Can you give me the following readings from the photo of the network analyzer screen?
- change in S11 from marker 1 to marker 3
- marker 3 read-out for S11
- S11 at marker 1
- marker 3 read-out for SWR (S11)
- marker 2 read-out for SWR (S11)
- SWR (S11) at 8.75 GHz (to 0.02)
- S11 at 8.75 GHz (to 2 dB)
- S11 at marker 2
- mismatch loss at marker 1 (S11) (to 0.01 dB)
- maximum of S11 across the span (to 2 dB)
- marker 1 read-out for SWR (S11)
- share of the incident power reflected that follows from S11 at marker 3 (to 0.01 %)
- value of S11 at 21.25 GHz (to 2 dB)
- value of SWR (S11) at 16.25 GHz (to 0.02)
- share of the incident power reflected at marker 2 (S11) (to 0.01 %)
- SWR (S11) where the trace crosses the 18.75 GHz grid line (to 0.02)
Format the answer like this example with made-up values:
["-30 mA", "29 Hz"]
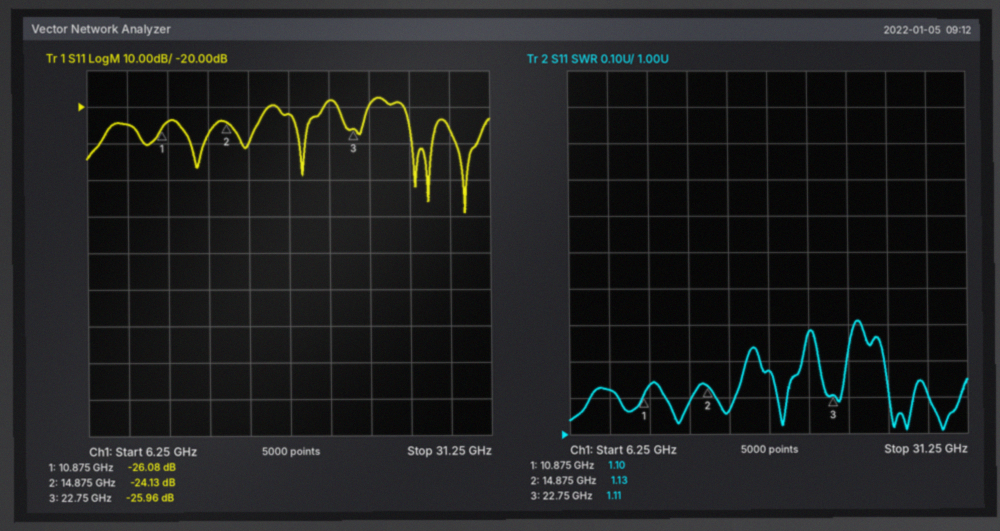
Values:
["0.12 dB", "-25.96 dB", "-26.08 dB", "1.11", "1.13", "1.12", "-24 dB", "-24.13 dB", "0.01 dB", "-18 dB", "1.10", "0.25 %", "-18 dB", "1.06", "0.39 %", "1.18"]
